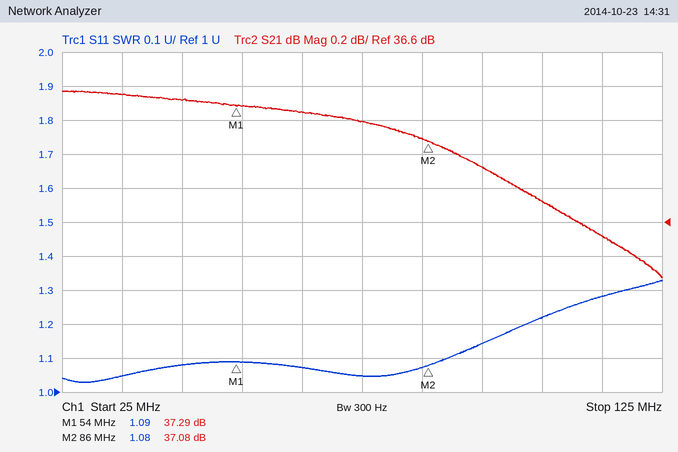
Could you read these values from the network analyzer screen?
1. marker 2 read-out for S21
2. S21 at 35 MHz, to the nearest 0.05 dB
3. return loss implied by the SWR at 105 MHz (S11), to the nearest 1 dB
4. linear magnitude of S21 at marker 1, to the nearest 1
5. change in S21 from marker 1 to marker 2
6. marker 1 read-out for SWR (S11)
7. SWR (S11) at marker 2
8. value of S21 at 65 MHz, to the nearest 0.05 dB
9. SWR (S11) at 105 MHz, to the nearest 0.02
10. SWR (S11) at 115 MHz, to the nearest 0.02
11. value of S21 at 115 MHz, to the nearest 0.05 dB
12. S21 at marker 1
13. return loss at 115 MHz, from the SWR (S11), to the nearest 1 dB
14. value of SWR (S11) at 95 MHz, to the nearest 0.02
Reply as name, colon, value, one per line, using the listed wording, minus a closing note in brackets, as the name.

marker 2 read-out for S21: 37.08 dB
S21 at 35 MHz, to the nearest 0.05 dB: 37.35 dB
return loss implied by the SWR at 105 MHz (S11), to the nearest 1 dB: 20 dB
linear magnitude of S21 at marker 1, to the nearest 1: 73
change in S21 from marker 1 to marker 2: -0.21 dB
marker 1 read-out for SWR: 1.09
SWR (S11) at marker 2: 1.08
value of S21 at 65 MHz, to the nearest 0.05 dB: 37.25 dB
SWR (S11) at 105 MHz, to the nearest 0.02: 1.22
SWR (S11) at 115 MHz, to the nearest 0.02: 1.28
value of S21 at 115 MHz, to the nearest 0.05 dB: 36.50 dB
S21 at marker 1: 37.29 dB
return loss at 115 MHz, from the SWR (S11), to the nearest 1 dB: 18 dB
value of SWR (S11) at 95 MHz, to the nearest 0.02: 1.14
